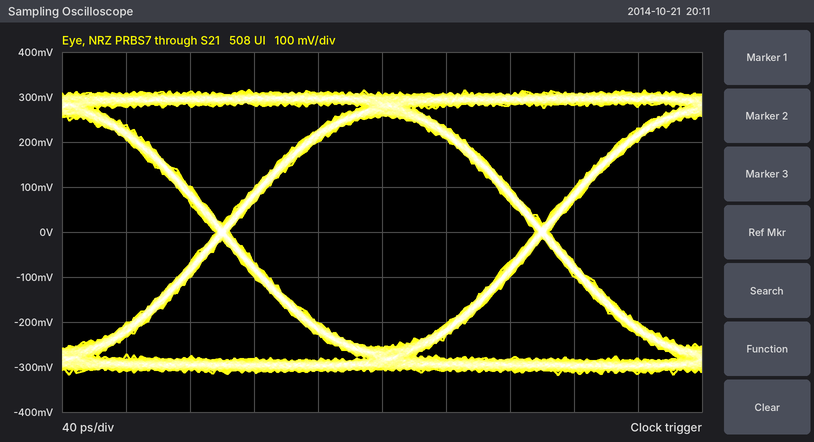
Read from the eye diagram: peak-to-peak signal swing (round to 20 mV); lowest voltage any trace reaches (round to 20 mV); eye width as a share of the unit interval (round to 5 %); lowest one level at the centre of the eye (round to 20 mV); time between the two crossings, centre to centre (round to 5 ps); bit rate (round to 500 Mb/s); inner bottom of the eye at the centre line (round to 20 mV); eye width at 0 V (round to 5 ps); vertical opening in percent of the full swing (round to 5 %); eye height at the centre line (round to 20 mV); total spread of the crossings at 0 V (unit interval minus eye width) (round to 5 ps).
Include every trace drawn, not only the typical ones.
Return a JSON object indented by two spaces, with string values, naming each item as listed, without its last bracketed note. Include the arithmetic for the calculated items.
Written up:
{
  "peak-to-peak signal swing": "640 mV",
  "lowest voltage any trace reaches": "-320 mV",
  "eye width as a share of the unit interval": "190 ps / 200 ps ≈ 95 %",
  "lowest one level at the centre of the eye": "260 mV",
  "time between the two crossings, centre to centre": "200 ps",
  "bit rate": "5.0 Gb/s",
  "inner bottom of the eye at the centre line": "-260 mV",
  "eye width at 0 V": "190 ps",
  "vertical opening in percent of the full swing": "520 mV / 640 mV ≈ 81.2 %, so 80 % to the nearest 5 %",
  "eye height at the centre line": "520 mV",
  "total spread of the crossings at 0 V (unit interval minus eye width)": "10 ps"
}
